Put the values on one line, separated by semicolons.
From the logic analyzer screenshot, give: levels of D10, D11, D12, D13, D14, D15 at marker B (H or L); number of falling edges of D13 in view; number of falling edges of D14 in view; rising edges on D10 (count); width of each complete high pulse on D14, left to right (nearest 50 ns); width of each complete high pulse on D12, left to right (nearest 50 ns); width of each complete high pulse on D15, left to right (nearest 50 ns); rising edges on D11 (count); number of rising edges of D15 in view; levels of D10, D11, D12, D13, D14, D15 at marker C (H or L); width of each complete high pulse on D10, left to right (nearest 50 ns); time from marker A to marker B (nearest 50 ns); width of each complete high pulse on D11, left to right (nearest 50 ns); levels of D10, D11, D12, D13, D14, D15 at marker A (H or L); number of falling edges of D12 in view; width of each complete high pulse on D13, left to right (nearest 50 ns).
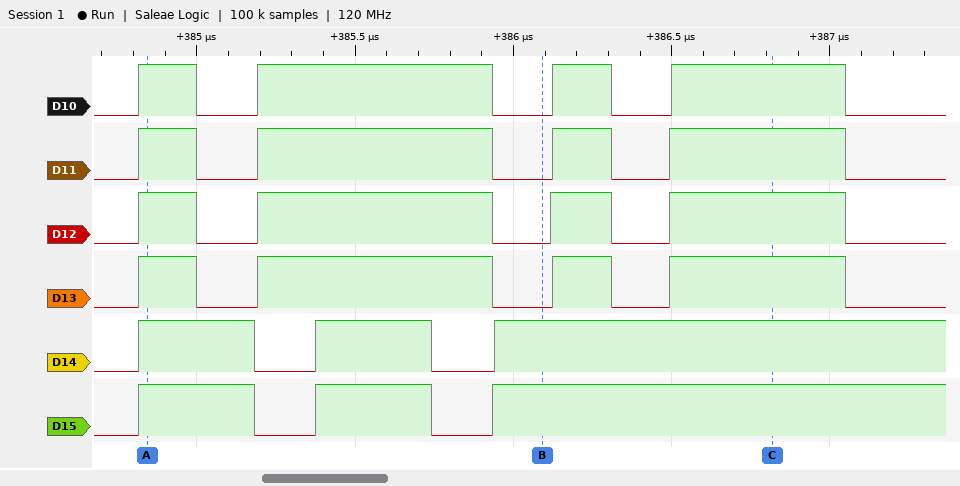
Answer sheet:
D10=L, D11=L, D12=L, D13=L, D14=H, D15=H; 4; 2; 4; 350 ns, 350 ns; 200 ns, 750 ns, 200 ns, 550 ns; 350 ns, 350 ns; 4; 3; D10=H, D11=H, D12=H, D13=H, D14=H, D15=H; 200 ns, 750 ns, 200 ns, 550 ns; 1250 ns; 200 ns, 750 ns, 200 ns, 550 ns; D10=H, D11=H, D12=H, D13=H, D14=H, D15=H; 4; 200 ns, 750 ns, 200 ns, 550 ns
